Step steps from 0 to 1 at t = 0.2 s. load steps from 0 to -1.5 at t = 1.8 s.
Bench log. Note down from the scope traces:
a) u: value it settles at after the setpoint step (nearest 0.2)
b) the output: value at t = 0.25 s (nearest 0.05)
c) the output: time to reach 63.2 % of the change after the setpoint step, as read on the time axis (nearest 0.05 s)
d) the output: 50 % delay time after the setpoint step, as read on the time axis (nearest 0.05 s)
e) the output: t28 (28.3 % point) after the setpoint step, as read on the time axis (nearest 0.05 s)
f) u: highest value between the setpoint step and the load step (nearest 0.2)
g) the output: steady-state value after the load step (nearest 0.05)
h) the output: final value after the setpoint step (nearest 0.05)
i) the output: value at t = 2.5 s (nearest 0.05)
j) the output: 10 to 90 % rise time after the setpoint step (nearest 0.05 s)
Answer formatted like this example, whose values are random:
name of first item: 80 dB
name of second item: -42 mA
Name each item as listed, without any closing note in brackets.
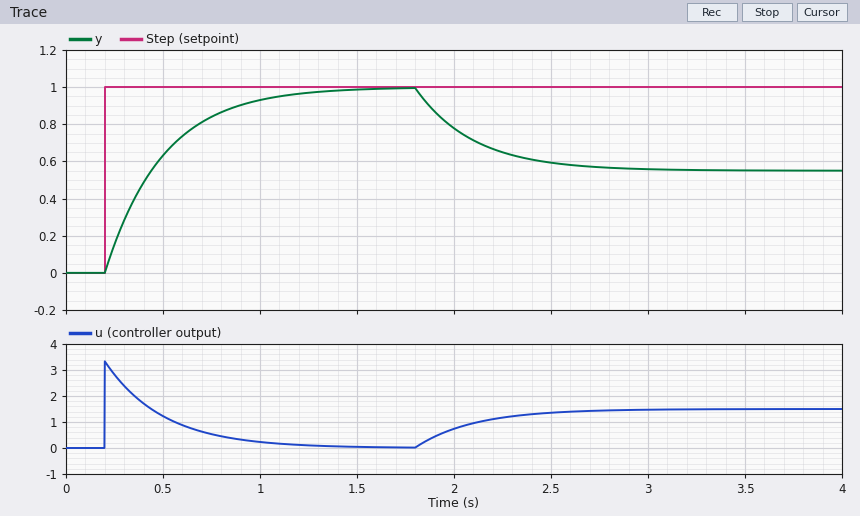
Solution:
u: value it settles at after the setpoint step: 0.0
the output: value at t = 0.25 s: 0.15
the output: time to reach 63.2 % of the change after the setpoint step, as read on the time axis: 0.50 s
the output: 50 % delay time after the setpoint step, as read on the time axis: 0.40 s
the output: t28 (28.3 % point) after the setpoint step, as read on the time axis: 0.30 s
u: highest value between the setpoint step and the load step: 3.4
the output: steady-state value after the load step: 0.55
the output: final value after the setpoint step: 1.00
the output: value at t = 2.5 s: 0.60
the output: 10 to 90 % rise time after the setpoint step: 0.65 s
